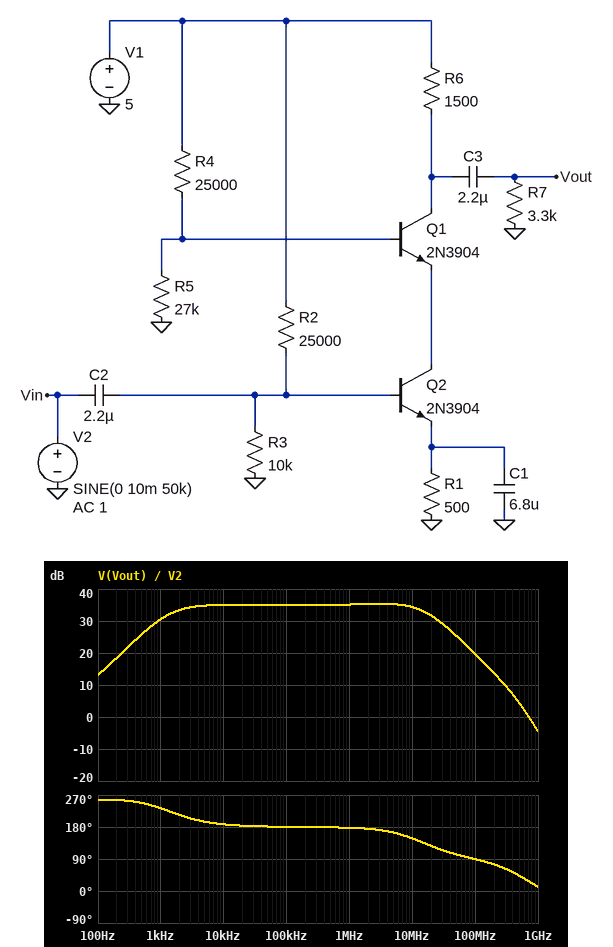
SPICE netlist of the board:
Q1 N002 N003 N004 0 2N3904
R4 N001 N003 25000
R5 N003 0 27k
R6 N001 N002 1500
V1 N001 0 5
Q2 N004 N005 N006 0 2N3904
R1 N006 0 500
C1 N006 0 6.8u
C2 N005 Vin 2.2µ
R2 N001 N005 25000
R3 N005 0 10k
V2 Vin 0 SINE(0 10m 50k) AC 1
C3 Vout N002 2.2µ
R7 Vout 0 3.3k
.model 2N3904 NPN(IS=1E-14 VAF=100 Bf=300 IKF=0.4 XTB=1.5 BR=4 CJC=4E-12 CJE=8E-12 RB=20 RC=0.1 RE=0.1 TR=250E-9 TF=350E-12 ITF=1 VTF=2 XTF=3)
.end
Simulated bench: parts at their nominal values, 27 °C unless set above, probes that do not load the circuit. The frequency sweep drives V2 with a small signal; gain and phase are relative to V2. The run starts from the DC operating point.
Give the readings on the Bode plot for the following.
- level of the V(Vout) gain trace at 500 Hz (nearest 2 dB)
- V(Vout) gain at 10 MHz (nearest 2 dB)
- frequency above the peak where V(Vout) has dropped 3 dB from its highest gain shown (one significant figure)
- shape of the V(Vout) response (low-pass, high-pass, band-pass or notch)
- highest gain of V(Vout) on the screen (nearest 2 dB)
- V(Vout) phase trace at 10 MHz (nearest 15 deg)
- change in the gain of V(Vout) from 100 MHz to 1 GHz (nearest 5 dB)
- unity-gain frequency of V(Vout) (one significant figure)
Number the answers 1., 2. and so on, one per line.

1. 26 dB
2. 34 dB
3. 20 MHz
4. band-pass
5. 36 dB
6. 150 deg
7. -25 dB
8. 700 MHz
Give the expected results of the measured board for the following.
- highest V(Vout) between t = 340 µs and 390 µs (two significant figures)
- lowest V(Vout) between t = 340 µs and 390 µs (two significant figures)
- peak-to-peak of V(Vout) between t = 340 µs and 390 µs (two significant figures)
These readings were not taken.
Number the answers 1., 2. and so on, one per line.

1. 510 mV
2. -620 mV
3. 1.1 V
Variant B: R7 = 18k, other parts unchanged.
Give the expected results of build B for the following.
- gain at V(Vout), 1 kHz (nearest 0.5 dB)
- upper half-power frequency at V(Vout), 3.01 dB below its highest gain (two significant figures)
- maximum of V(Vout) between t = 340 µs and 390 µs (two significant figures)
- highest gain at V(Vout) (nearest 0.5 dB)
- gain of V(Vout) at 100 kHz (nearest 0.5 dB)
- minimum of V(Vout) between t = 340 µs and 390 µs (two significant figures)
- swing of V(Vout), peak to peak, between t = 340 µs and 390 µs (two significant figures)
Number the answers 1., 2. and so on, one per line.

1. 33.0 dB
2. 14 MHz
3. 680 mV
4. 38.0 dB
5. 37.5 dB
6. -830 mV
7. 1.5 V
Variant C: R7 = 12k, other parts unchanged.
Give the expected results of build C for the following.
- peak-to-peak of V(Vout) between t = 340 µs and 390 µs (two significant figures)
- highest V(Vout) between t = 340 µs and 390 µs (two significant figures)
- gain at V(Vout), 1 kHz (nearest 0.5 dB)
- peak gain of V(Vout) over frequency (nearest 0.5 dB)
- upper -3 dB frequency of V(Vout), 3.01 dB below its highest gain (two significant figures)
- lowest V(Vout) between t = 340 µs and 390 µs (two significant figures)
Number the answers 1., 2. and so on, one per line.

1. 1.5 V
2. 660 mV
3. 33.0 dB
4. 37.5 dB
5. 15 MHz
6. -800 mV
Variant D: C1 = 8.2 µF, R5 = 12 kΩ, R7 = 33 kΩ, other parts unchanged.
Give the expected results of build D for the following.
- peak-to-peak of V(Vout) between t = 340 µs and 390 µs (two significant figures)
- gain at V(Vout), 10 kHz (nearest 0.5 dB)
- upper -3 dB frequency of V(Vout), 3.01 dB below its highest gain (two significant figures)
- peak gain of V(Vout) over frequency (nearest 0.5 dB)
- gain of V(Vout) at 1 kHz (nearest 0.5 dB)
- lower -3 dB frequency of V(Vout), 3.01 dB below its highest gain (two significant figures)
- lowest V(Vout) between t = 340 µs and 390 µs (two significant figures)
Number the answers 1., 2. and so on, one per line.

1. 1.6 V
2. 38.0 dB
3. 5.9 MHz
4. 40.5 dB
5. 34.5 dB
6. 4.1 kHz
7. -860 mV
